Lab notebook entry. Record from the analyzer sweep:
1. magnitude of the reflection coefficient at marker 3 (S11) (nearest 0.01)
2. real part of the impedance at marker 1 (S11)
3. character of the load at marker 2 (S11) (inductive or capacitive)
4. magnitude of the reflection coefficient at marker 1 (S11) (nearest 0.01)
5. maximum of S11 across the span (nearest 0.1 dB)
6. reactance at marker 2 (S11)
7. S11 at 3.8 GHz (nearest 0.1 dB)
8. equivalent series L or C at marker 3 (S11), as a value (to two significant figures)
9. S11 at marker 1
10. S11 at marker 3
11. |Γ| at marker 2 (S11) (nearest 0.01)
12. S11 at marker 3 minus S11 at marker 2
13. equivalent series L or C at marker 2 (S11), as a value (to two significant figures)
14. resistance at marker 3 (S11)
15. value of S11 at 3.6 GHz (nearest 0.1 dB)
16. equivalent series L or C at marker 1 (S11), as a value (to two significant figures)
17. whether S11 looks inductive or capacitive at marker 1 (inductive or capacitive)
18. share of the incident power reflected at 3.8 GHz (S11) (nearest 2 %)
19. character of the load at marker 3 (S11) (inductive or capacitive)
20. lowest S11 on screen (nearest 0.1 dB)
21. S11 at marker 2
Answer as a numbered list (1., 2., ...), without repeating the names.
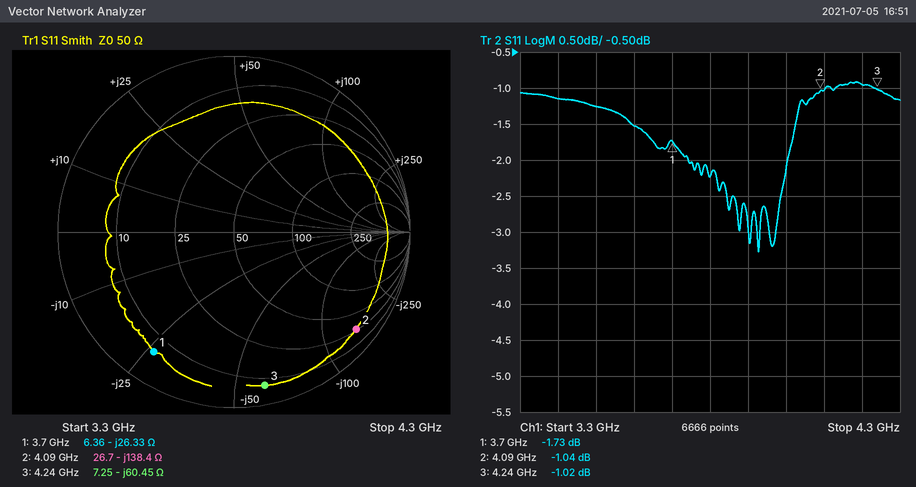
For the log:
1. 0.89
2. 6.36 Ω
3. capacitive
4. 0.82
5. -0.9 dB
6. -138.4 Ω
7. -2.2 dB
8. 620 fF
9. -1.73 dB
10. -1.02 dB
11. 0.89
12. 0.02 dB
13. 280 fF
14. 7.25 Ω
15. -1.5 dB
16. 1.6 pF
17. capacitive
18. 60 %
19. capacitive
20. -3.3 dB
21. -1.04 dB
